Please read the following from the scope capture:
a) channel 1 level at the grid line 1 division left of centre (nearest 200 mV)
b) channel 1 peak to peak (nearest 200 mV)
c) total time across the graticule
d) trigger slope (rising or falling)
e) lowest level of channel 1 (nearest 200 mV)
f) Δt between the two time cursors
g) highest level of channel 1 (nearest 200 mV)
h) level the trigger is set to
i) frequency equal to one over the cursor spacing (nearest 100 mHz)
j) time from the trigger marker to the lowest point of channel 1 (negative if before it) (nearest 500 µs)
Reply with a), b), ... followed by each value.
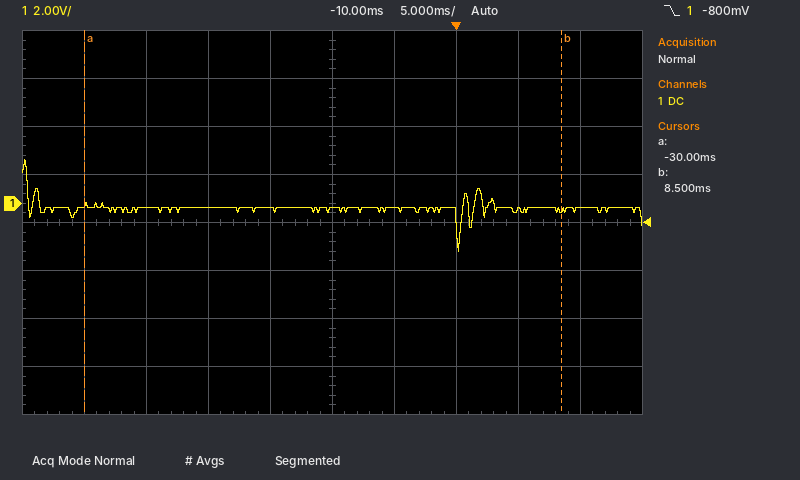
a) -200 mV
b) 3.8 V
c) 50 ms
d) falling
e) -2.0 V
f) 38.5 ms
g) 1.8 V
h) -800 mV
i) 26.0 Hz
j) 0.0 ms
